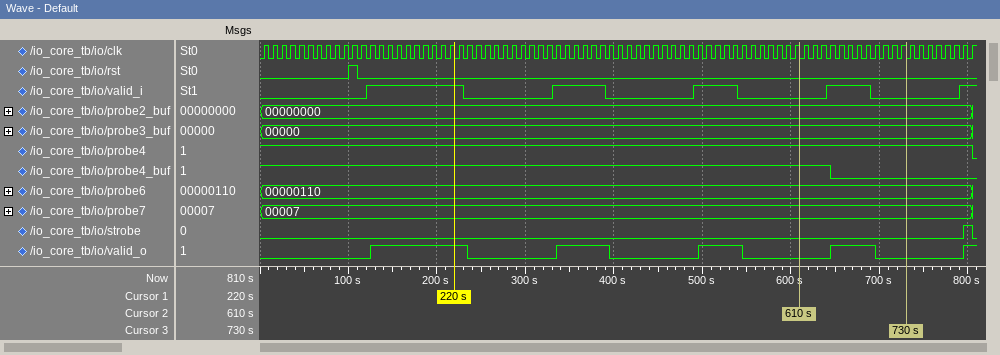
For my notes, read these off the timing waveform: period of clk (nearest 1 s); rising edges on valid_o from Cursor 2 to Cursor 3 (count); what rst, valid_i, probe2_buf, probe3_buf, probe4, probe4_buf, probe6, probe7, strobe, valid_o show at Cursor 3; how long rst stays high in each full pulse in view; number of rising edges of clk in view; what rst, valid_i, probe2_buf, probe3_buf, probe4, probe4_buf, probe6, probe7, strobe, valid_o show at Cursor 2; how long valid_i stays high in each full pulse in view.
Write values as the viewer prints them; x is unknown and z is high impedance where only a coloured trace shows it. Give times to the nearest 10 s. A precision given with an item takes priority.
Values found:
10 s
1
rst=0, valid_i=0, probe2_buf=00000000, probe3_buf=00000, probe4=1, probe4_buf=0, probe6=00000110, probe7=00007, strobe=0, valid_o=0
10 s
81
rst=0, valid_i=0, probe2_buf=00000000, probe3_buf=00000, probe4=1, probe4_buf=1, probe6=00000110, probe7=00007, strobe=0, valid_o=0
110 s, 60 s, 50 s, 50 s
